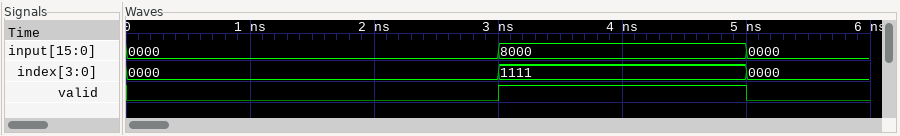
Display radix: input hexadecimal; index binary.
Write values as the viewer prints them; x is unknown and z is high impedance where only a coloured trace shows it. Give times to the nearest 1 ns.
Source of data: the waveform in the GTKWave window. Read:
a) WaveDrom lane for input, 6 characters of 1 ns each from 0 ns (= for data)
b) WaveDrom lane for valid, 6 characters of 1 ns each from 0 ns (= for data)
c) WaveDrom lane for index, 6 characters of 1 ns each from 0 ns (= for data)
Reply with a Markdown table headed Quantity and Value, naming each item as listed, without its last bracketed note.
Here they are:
| Quantity | Value |
|---|---|
| WaveDrom lane for input, 6 characters of 1 ns each from 0 ns | {name: 'input', wave: '=..=.=', data: '0000 8000 0000'} |
| WaveDrom lane for valid, 6 characters of 1 ns each from 0 ns | {name: 'valid', wave: '0..1.0'} |
| WaveDrom lane for index, 6 characters of 1 ns each from 0 ns | {name: 'index', wave: '=..=.=', data: '0000 1111 0000'} |
